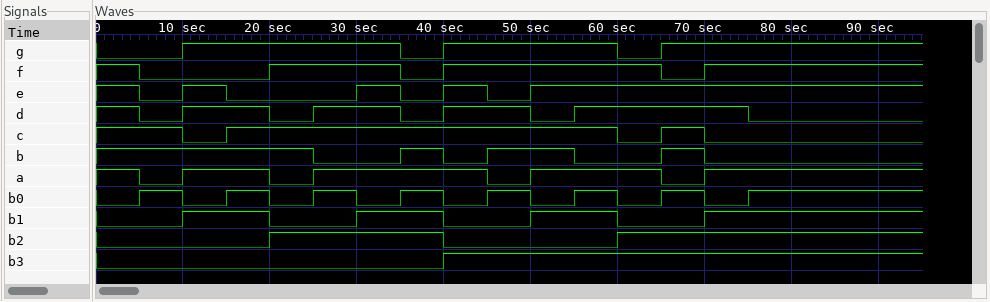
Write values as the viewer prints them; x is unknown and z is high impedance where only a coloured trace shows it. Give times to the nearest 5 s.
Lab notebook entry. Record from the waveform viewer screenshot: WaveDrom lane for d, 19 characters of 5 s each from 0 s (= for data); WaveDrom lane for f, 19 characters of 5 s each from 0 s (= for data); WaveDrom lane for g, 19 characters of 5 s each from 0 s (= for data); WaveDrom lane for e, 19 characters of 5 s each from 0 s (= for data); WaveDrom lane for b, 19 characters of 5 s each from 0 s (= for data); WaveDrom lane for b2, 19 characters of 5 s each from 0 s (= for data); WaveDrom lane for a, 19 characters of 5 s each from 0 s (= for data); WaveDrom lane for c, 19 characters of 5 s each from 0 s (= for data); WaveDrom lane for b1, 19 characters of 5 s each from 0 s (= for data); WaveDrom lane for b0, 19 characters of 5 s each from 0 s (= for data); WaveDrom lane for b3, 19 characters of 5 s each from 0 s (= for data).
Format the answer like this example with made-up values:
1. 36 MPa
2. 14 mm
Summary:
1. {name: 'd', wave: '101.01.01.01...0...'}
2. {name: 'f', wave: '10..1..01....01....'}
3. {name: 'g', wave: '0.1....01...01.....'}
4. {name: 'e', wave: '1010..10101........'}
5. {name: 'b', wave: '1....0.101.0.10....'}
6. {name: 'b2', wave: '0...1...0...1......'}
7. {name: 'a', wave: '101.01...01..01....'}
8. {name: 'c', wave: '1.01........010....'}
9. {name: 'b1', wave: '0.1.0.1.0.1.0.1....'}
10. {name: 'b0', wave: '0101010101010101...'}
11. {name: 'b3', wave: '0.......1..........'}
